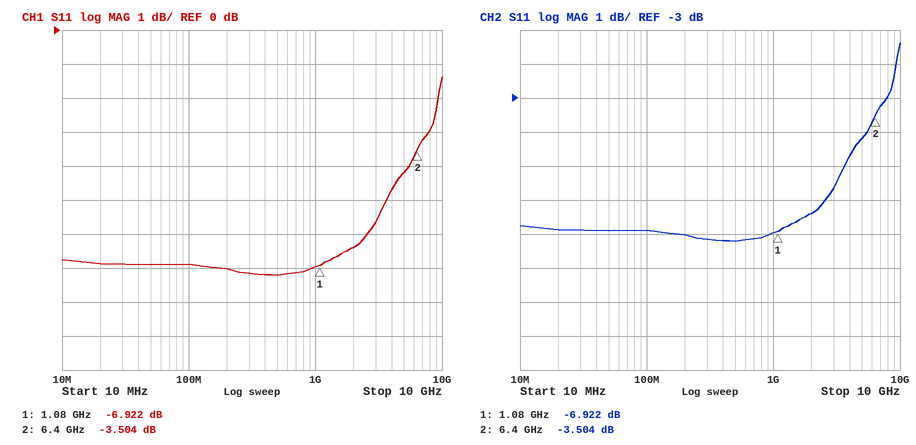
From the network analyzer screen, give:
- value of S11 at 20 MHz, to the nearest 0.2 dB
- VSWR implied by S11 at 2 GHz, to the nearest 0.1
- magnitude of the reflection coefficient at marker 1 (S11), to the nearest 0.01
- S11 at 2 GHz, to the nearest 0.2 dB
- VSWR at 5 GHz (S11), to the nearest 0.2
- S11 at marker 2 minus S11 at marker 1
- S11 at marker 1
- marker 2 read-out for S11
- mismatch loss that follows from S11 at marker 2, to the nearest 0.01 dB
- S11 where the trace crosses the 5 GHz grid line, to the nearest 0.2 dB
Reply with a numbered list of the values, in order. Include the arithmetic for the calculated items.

1. -6.8 dB
2. |Γ| = 10^(-6.4/20) = 0.4786; VSWR = (1 + 0.4786)/(1 − 0.4786) ≈ 2.8
3. 10^(-6.922/20) ≈ 0.45
4. -6.4 dB
5. |Γ| = 10^(-4.2/20) = 0.6166; VSWR = (1 + 0.6166)/(1 − 0.6166) ≈ 4.2
6. -3.504 − (-6.922) = 3.418 dB
7. -6.922 dB
8. -3.504 dB
9. −10 log10(1 − 10^(-3.504/10)) ≈ 2.57 dB
10. -4.2 dB
